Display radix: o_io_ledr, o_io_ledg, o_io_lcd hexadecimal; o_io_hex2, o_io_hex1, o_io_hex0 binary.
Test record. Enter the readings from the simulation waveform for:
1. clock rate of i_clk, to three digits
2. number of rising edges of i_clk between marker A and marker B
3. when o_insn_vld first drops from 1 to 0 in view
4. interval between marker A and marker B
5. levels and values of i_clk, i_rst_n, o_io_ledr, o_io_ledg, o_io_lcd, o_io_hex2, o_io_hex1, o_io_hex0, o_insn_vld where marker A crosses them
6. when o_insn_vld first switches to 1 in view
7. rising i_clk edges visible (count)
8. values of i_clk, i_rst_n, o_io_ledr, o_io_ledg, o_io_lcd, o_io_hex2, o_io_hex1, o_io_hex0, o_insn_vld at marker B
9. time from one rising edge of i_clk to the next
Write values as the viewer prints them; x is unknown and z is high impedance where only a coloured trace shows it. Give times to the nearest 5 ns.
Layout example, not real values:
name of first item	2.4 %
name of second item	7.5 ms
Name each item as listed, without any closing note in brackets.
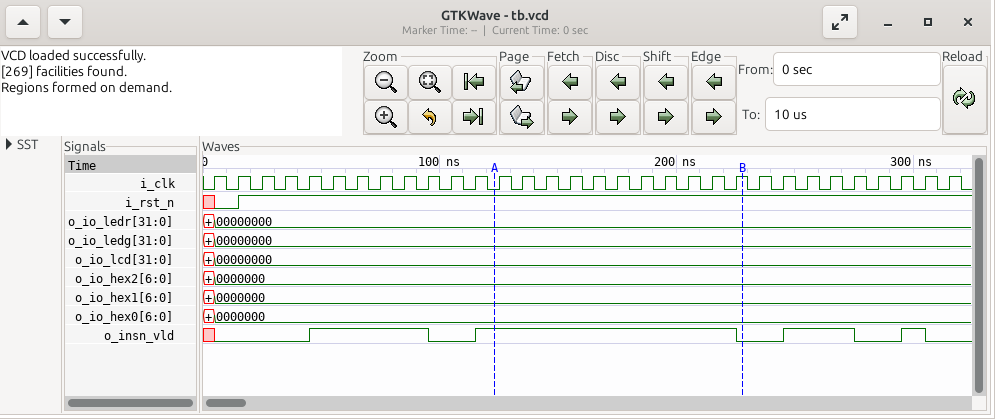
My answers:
clock rate of i_clk, to three digits	100 MHz
number of rising edges of i_clk between marker A and marker B	11
when o_insn_vld first drops from 1 to 0 in view	95 ns
interval between marker A and marker B	105 ns
levels and values of i_clk, i_rst_n, o_io_ledr, o_io_ledg, o_io_lcd, o_io_hex2, o_io_hex1, o_io_hex0, o_insn_vld where marker A crosses them	i_clk=0, i_rst_n=1, o_io_ledr=00000000, o_io_ledg=00000000, o_io_lcd=00000000, o_io_hex2=0000000, o_io_hex1=0000000, o_io_hex0=0000000, o_insn_vld=1
when o_insn_vld first switches to 1 in view	45 ns
rising i_clk edges visible	32
values of i_clk, i_rst_n, o_io_ledr, o_io_ledg, o_io_lcd, o_io_hex2, o_io_hex1, o_io_hex0, o_insn_vld at marker B	i_clk=1, i_rst_n=1, o_io_ledr=00000000, o_io_ledg=00000000, o_io_lcd=00000000, o_io_hex2=0000000, o_io_hex1=0000000, o_io_hex0=0000000, o_insn_vld=0
time from one rising edge of i_clk to the next	10 ns
